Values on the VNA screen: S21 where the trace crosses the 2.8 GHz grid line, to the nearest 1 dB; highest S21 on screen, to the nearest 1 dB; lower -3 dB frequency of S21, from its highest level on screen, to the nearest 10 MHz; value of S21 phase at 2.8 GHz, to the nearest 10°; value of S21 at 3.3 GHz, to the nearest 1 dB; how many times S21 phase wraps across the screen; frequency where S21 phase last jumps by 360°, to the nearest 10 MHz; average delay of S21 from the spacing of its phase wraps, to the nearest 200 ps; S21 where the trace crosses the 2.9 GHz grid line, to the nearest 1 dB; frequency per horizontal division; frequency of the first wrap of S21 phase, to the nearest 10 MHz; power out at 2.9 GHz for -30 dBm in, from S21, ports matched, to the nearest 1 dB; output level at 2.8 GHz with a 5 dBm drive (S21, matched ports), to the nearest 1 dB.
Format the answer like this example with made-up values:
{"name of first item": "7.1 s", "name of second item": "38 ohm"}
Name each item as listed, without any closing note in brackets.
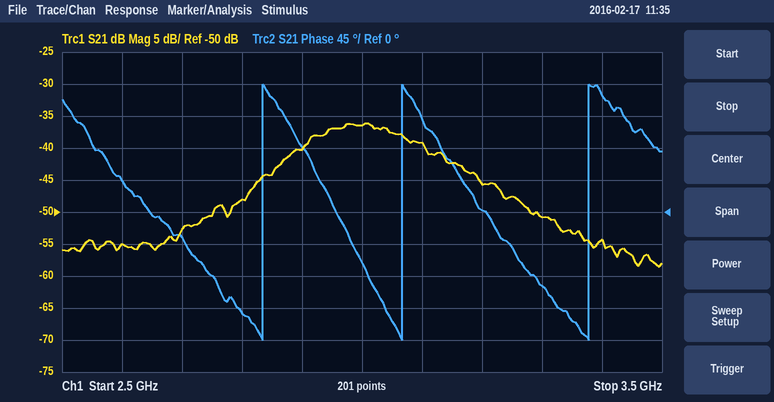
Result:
{"S21 where the trace crosses the 2.8 GHz grid line, to the nearest 1 dB": "-48 dB", "highest S21 on screen, to the nearest 1 dB": "-36 dB", "lower -3 dB frequency of S21, from its highest level on screen, to the nearest 10 MHz": "2.91 GHz", "value of S21 phase at 2.8 GHz, to the nearest 10°": "-140°", "value of S21 at 3.3 GHz, to the nearest 1 dB": "-51 dB", "how many times S21 phase wraps across the screen": "3", "frequency where S21 phase last jumps by 360°, to the nearest 10 MHz": "3.38 GHz", "average delay of S21 from the spacing of its phase wraps, to the nearest 200 ps": "3.6 ns", "S21 where the trace crosses the 2.9 GHz grid line, to the nearest 1 dB": "-40 dB", "frequency per horizontal division": "100 MHz", "frequency of the first wrap of S21 phase, to the nearest 10 MHz": "2.83 GHz", "power out at 2.9 GHz for -30 dBm in, from S21, ports matched, to the nearest 1 dB": "-70 dBm", "output level at 2.8 GHz with a 5 dBm drive (S21, matched ports), to the nearest 1 dB": "-43 dBm"}
